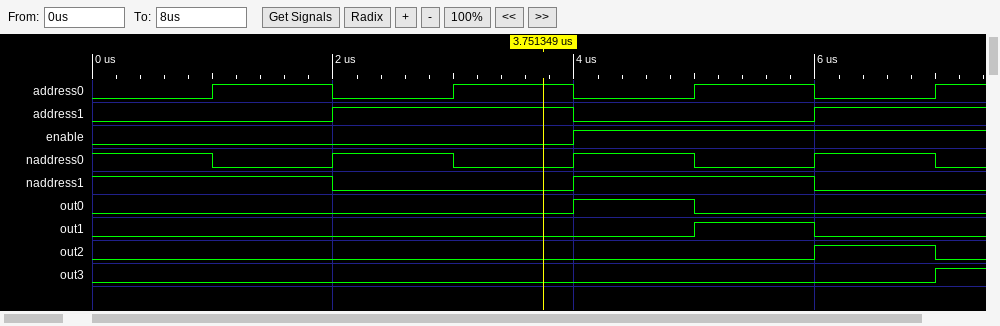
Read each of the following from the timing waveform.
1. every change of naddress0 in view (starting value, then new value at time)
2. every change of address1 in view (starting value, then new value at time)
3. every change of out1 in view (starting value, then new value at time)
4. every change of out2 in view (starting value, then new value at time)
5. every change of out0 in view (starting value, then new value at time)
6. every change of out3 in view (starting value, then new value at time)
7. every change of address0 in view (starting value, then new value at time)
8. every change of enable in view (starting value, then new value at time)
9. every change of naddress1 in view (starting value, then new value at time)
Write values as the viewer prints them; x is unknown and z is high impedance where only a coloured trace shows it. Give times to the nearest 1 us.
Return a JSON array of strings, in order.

["1, 0 at 1 us, 1 at 2 us, 0 at 3 us, 1 at 4 us, 0 at 5 us, 1 at 6 us, 0 at 7 us", "0, 1 at 2 us, 0 at 4 us, 1 at 6 us", "0, 1 at 5 us, 0 at 6 us", "0, 1 at 6 us, 0 at 7 us", "0, 1 at 4 us, 0 at 5 us", "0, 1 at 7 us", "0, 1 at 1 us, 0 at 2 us, 1 at 3 us, 0 at 4 us, 1 at 5 us, 0 at 6 us, 1 at 7 us", "0, 1 at 4 us", "1, 0 at 2 us, 1 at 4 us, 0 at 6 us"]
